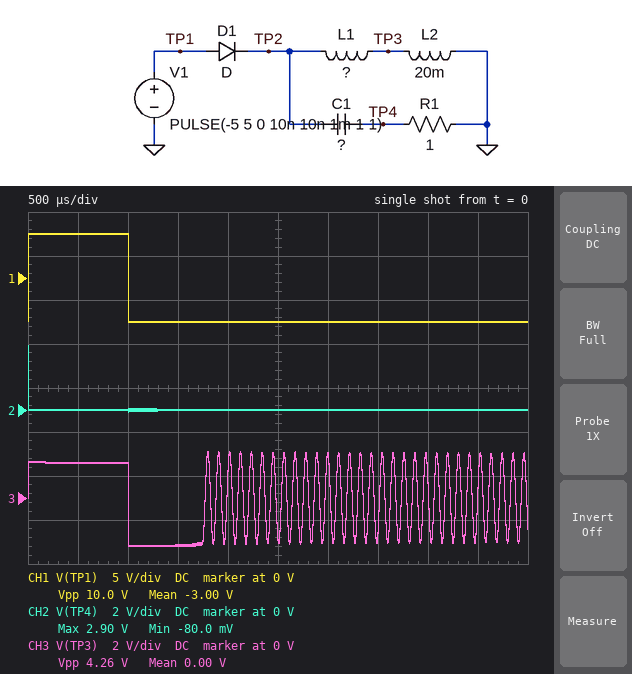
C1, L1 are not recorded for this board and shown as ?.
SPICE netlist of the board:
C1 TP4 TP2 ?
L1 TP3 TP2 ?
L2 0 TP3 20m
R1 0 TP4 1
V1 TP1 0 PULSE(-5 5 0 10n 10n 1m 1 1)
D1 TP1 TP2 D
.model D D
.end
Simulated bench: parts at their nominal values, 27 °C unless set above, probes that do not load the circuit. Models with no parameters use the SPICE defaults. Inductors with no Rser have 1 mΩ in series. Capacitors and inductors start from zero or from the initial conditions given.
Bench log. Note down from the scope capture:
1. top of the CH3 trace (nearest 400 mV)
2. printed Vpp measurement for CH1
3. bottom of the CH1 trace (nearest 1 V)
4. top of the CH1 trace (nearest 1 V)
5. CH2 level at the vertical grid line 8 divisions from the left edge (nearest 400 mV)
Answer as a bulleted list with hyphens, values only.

- 2.0 V
- 10.0 V
- -5 V
- 5 V
- 0 V
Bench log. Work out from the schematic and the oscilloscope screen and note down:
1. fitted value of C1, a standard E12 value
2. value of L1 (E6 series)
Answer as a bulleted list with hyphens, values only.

- 5.6 nF
- 33 mH
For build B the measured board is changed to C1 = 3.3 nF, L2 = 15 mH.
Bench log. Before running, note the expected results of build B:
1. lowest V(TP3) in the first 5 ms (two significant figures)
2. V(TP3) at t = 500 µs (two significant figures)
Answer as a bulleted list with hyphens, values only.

- -1.8 V
- 1.3 V
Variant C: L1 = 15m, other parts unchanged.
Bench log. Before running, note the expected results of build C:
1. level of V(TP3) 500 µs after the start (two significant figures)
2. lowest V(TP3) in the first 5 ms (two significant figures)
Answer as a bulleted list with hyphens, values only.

- 2.4 V
- -3.3 V
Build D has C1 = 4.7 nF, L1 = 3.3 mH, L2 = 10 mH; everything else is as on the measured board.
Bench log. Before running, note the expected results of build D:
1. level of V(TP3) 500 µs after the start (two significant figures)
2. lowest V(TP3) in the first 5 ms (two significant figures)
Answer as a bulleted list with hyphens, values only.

- 3.2 V
- -4.4 V
